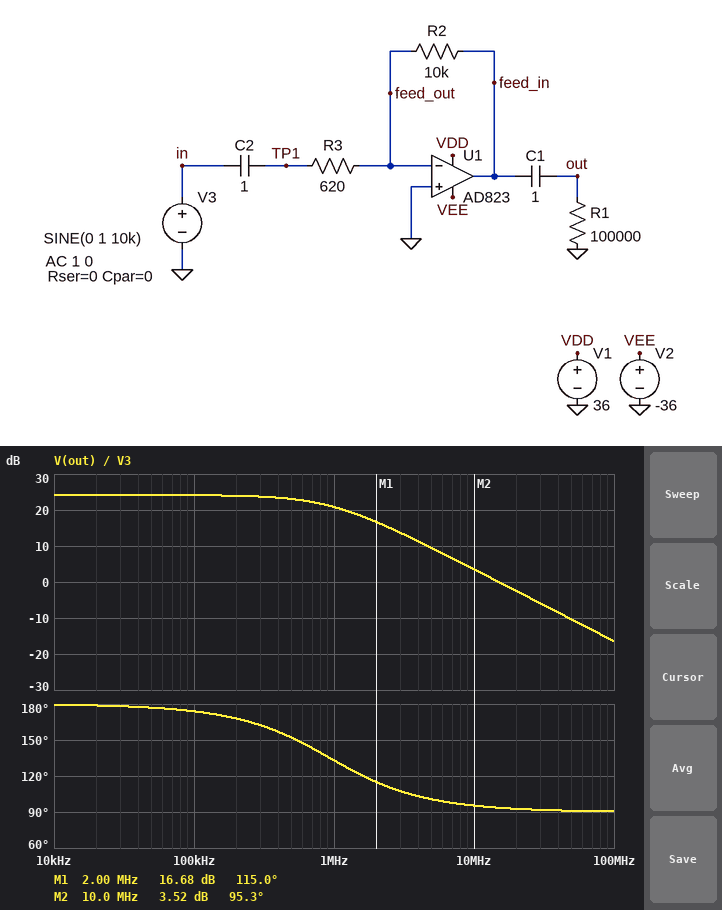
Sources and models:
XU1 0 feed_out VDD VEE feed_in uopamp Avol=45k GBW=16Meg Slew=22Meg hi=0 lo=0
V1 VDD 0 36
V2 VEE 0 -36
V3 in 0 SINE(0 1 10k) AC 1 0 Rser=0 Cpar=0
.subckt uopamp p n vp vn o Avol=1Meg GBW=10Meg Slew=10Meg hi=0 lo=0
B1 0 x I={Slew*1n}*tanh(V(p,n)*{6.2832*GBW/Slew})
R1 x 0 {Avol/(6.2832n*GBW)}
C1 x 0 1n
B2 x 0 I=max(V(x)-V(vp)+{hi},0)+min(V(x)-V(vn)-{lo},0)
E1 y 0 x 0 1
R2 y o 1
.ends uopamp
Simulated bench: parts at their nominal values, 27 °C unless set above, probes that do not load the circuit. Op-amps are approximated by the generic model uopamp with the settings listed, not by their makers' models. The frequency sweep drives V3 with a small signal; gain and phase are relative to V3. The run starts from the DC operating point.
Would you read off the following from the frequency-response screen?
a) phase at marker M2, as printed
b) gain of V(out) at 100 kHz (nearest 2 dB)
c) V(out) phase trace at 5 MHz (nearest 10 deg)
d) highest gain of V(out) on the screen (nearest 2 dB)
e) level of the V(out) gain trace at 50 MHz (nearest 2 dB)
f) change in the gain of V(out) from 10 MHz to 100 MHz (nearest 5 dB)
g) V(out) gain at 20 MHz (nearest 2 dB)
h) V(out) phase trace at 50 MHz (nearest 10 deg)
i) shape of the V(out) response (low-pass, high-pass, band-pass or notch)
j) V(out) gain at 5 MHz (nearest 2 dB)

95.3 deg
24 dB
100 deg
24 dB
-10 dB
-20 dB
-2 dB
90 deg
low-pass
10 dB
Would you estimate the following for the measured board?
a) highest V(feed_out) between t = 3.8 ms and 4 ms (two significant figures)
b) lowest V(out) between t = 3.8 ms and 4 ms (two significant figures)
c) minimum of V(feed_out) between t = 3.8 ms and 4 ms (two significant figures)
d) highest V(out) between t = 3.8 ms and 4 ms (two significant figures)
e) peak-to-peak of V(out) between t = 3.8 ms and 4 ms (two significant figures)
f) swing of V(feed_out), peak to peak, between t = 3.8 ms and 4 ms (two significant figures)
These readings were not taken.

10 mV
-16 V
-10 mV
16 V
32 V
20 mV
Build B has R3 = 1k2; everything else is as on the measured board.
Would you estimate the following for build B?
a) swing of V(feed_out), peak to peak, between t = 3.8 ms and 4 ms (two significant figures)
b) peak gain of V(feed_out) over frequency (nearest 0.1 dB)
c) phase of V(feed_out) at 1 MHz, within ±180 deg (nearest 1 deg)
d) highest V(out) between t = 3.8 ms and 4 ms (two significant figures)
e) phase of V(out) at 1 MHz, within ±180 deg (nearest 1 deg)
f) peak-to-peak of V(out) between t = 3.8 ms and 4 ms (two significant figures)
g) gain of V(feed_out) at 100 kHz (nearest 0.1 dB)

10 mV
-1.0 dB
60 deg
8.3 V
150 deg
17 V
-25.7 dB
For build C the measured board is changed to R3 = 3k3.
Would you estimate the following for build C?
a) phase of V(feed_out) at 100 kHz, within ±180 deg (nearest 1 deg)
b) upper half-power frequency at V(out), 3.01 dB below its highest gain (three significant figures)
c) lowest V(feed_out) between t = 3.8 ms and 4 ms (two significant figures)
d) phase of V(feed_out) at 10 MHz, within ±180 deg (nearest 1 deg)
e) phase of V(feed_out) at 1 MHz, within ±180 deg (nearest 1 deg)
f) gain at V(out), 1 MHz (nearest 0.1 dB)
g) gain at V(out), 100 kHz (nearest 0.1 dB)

88 deg
3.97 MHz
-1.9 mV
22 deg
76 deg
9.4 dB
9.6 dB
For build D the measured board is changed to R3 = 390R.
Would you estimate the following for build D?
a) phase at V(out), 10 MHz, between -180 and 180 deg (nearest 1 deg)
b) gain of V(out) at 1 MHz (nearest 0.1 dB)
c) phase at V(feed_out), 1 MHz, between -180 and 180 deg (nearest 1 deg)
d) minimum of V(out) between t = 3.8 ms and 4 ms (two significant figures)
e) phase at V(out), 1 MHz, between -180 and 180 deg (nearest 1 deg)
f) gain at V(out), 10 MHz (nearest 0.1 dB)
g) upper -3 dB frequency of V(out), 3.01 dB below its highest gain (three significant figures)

93 deg
22.4 dB
31 deg
-26 V
121 deg
3.7 dB
601 kHz
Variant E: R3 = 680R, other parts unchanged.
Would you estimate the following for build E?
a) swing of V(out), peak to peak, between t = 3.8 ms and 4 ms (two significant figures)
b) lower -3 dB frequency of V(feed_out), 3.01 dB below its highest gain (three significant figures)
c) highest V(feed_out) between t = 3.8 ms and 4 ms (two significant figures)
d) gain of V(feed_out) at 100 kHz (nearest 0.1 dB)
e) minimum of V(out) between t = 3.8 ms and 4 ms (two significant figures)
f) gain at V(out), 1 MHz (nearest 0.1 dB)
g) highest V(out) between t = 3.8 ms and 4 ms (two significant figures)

29 V
1.02 MHz
9.2 mV
-20.8 dB
-15 V
20.4 dB
15 V
